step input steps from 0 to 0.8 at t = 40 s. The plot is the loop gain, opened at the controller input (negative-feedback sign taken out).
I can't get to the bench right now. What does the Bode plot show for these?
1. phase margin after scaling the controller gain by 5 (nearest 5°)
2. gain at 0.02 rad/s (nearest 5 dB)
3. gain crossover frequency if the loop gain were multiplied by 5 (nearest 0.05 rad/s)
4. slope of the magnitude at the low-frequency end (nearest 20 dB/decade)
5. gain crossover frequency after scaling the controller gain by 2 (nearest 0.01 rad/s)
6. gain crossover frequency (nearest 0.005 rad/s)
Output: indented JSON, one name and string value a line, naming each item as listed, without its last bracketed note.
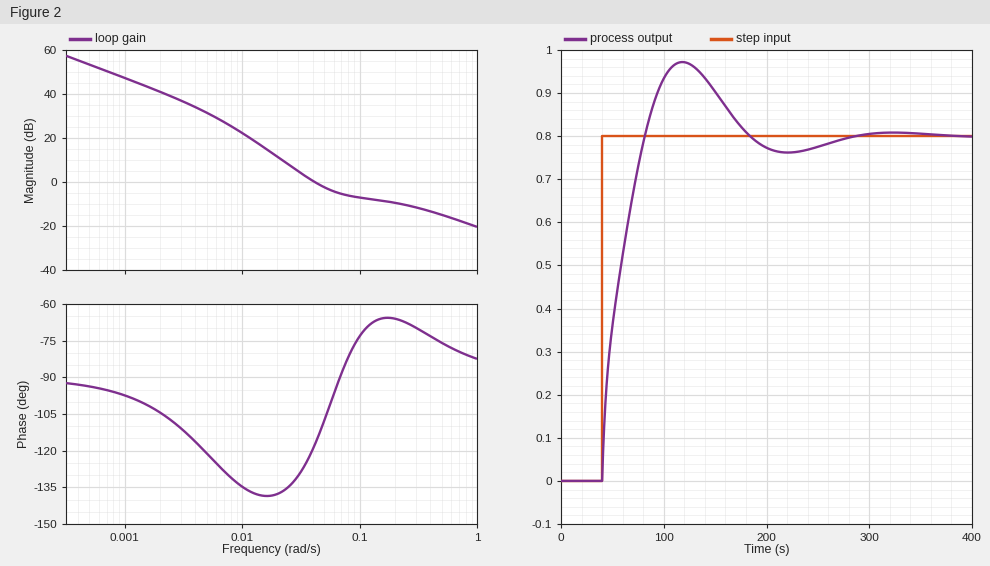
{
  "phase margin after scaling the controller gain by 5": "105°",
  "gain at 0.02 rad/s": "10 dB",
  "gain crossover frequency if the loop gain were multiplied by 5": "0.45 rad/s",
  "slope of the magnitude at the low-frequency end": "-20 dB/decade",
  "gain crossover frequency after scaling the controller gain by 2": "0.08 rad/s",
  "gain crossover frequency": "0.040 rad/s"
}
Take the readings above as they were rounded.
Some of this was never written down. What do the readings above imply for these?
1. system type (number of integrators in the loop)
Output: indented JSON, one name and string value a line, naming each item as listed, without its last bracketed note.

{
  "system type": "1"
}
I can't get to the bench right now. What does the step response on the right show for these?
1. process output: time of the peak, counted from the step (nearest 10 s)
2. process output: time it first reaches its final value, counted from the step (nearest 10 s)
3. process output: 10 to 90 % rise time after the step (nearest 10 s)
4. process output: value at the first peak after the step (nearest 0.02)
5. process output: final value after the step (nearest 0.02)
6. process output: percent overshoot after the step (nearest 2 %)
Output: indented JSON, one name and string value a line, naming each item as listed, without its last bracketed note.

{
  "process output: time of the peak, counted from the step": "80 s",
  "process output: time it first reaches its final value, counted from the step": "40 s",
  "process output: 10 to 90 % rise time after the step": "30 s",
  "process output: value at the first peak after the step": "0.98",
  "process output: final value after the step": "0.80",
  "process output: percent overshoot after the step": "22 %"
}
